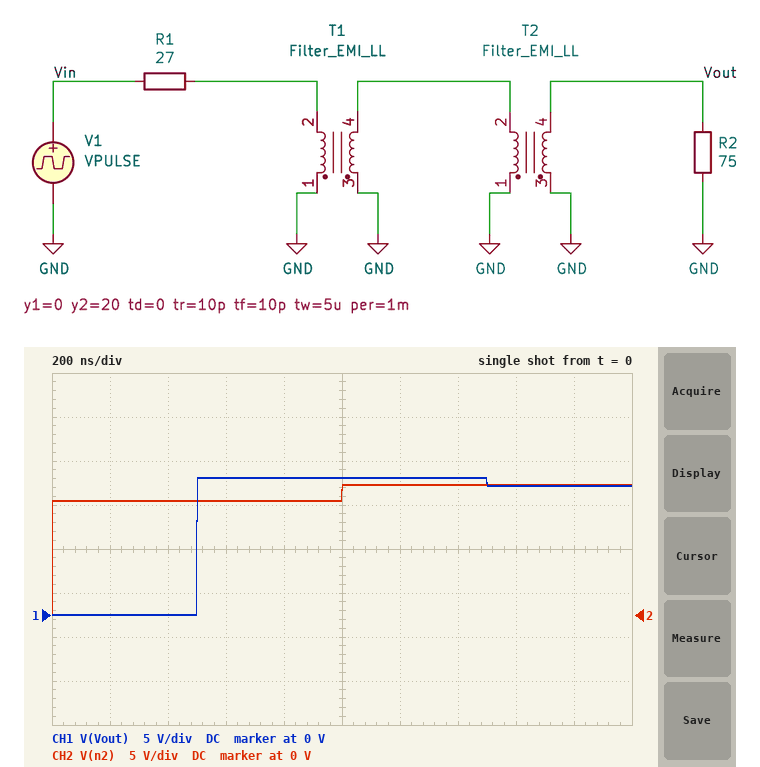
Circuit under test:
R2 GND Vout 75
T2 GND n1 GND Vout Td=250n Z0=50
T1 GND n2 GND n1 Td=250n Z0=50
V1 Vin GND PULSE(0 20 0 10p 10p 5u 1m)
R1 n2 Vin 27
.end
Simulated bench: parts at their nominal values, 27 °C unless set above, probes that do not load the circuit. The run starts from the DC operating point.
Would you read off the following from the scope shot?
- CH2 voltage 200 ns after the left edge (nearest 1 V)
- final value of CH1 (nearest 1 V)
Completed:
13 V
15 V
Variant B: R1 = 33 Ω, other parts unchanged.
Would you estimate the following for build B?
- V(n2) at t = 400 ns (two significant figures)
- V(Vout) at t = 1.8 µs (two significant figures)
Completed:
12 V
14 V
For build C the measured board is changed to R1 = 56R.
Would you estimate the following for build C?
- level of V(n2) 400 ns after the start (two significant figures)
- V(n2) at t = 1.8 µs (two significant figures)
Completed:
9.4 V
11 V
